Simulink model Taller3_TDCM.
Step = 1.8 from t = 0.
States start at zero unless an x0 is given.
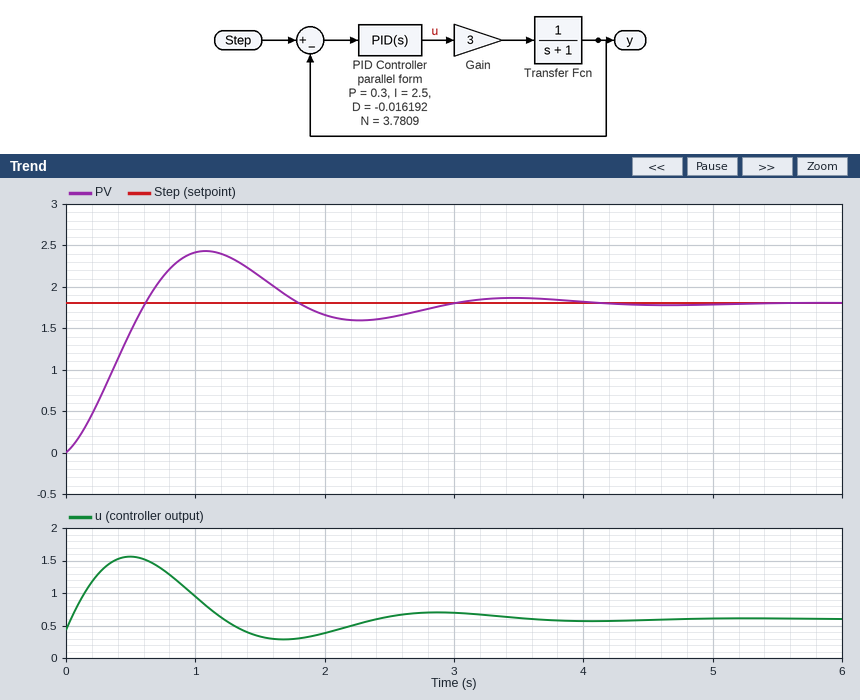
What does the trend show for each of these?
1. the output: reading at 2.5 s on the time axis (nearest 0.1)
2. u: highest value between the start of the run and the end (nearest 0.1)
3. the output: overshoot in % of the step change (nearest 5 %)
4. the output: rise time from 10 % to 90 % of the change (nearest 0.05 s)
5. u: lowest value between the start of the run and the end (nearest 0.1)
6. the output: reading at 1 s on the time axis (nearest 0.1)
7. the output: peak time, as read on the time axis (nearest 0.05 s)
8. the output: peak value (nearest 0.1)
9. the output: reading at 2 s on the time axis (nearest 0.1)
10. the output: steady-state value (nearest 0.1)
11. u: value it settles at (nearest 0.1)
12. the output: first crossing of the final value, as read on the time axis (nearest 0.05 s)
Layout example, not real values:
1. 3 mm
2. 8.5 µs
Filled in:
1. 1.6
2. 1.6
3. 35 %
4. 0.45 s
5. 0.3
6. 2.4
7. 1.10 s
8. 2.4
9. 1.7
10. 1.8
11. 0.6
12. 0.60 s
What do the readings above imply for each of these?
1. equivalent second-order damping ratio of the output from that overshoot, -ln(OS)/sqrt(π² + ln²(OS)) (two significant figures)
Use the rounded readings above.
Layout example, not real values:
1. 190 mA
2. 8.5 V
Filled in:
1. 0.32
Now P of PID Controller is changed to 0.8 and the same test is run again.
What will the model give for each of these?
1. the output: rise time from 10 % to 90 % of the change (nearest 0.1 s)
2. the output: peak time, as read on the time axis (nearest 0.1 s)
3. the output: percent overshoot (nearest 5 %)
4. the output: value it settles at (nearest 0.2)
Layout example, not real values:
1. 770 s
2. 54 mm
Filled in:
1. 0.4 s
2. 1.0 s
3. 15 %
4. 1.8
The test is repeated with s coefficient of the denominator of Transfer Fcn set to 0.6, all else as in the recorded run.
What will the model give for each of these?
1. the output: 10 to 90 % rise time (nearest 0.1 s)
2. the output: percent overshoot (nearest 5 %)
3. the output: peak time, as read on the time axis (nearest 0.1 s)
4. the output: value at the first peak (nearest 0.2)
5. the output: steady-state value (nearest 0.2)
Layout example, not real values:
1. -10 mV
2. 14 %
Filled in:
1. 0.4 s
2. 25 %
3. 0.8 s
4. 2.2
5. 1.8
